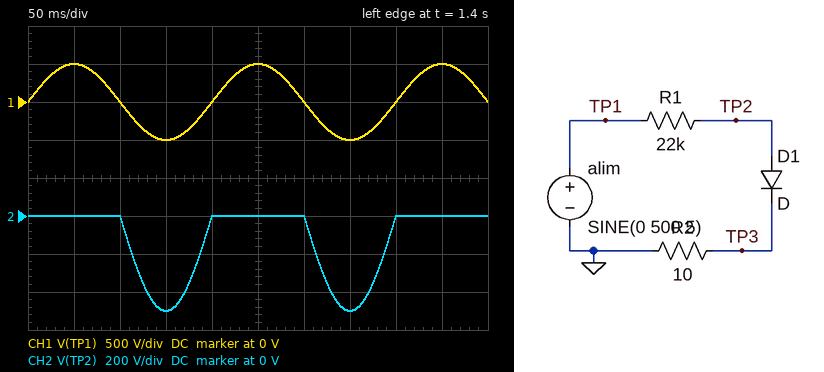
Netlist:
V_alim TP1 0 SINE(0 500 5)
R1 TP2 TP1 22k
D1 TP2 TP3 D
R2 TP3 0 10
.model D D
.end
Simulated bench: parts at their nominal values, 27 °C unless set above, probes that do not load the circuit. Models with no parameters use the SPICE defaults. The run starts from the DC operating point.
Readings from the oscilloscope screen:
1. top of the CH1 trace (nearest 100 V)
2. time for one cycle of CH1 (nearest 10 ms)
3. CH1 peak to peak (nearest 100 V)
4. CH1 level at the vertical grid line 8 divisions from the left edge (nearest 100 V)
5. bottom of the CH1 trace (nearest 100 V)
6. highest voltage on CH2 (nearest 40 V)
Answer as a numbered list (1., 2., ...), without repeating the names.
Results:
1. 500 V
2. 200 ms
3. 1.0 kV
4. 0 V
5. -500 V
6. 0 V
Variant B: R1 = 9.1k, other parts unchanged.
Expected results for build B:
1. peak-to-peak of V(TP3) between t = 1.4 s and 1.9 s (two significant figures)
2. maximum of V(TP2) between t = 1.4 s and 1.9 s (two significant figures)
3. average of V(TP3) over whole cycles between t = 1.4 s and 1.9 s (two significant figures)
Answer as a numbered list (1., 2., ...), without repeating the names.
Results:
1. 550 mV
2. 1.3 V
3. 170 mV
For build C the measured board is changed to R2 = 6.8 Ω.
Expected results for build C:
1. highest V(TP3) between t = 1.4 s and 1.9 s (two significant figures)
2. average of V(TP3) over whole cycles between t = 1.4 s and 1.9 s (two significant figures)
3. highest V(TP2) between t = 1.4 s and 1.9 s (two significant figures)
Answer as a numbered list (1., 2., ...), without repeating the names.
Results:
1. 150 mV
2. 49 mV
3. 890 mV
